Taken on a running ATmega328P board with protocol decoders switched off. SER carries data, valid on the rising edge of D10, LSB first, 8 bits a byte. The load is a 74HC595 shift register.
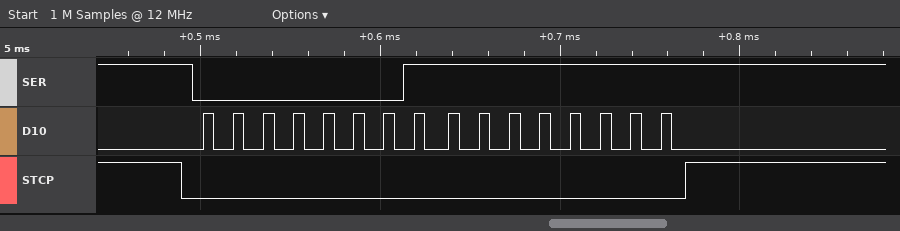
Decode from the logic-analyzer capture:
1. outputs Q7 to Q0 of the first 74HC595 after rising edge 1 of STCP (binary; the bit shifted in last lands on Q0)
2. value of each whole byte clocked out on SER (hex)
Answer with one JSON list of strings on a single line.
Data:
["11111111", "80 FF"]
